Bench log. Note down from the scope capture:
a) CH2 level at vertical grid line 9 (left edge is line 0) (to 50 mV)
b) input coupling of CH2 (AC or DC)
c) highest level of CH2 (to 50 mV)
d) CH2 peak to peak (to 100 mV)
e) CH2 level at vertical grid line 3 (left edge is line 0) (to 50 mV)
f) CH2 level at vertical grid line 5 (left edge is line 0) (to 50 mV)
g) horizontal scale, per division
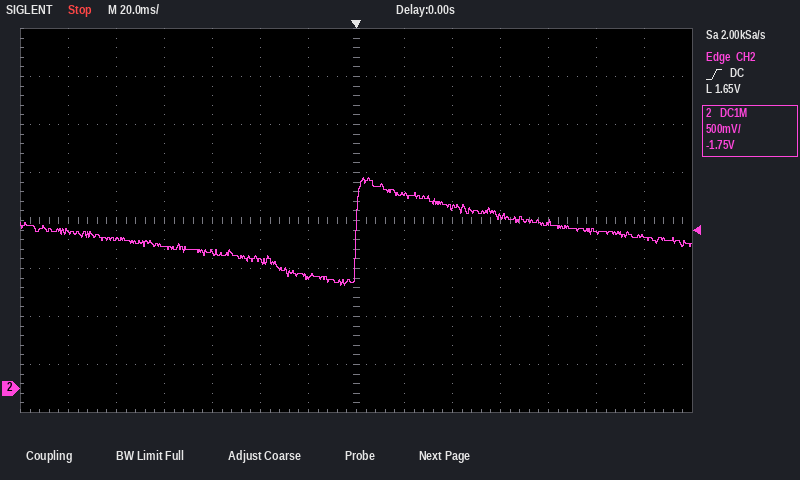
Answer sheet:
1.90 V
DC
2.20 V
1.10 V
1.50 V
1.35 V
20 ms
